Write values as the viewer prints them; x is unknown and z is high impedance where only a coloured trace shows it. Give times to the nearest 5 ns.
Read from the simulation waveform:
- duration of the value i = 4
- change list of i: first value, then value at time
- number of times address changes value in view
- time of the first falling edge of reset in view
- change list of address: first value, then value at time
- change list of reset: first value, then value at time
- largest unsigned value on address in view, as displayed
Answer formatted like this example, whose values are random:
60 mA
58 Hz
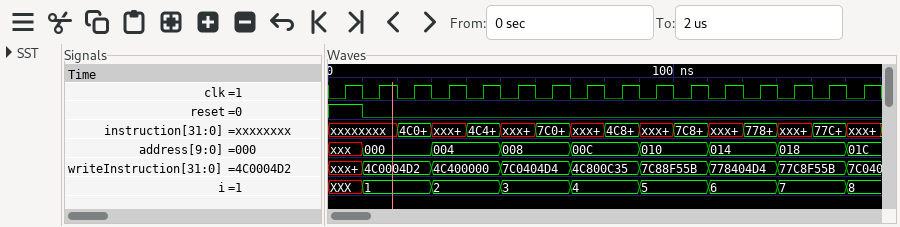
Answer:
20 ns
XXX, 1 at 10 ns, 2 at 30 ns, 3 at 50 ns, 4 at 70 ns, 5 at 90 ns, 6 at 110 ns, 7 at 130 ns, 8 at 150 ns
8
10 ns
xxx, 000 at 10 ns, 004 at 30 ns, 008 at 50 ns, 00C at 70 ns, 010 at 90 ns, 014 at 110 ns, 018 at 130 ns, 01C at 150 ns
1, 0 at 10 ns
01C
